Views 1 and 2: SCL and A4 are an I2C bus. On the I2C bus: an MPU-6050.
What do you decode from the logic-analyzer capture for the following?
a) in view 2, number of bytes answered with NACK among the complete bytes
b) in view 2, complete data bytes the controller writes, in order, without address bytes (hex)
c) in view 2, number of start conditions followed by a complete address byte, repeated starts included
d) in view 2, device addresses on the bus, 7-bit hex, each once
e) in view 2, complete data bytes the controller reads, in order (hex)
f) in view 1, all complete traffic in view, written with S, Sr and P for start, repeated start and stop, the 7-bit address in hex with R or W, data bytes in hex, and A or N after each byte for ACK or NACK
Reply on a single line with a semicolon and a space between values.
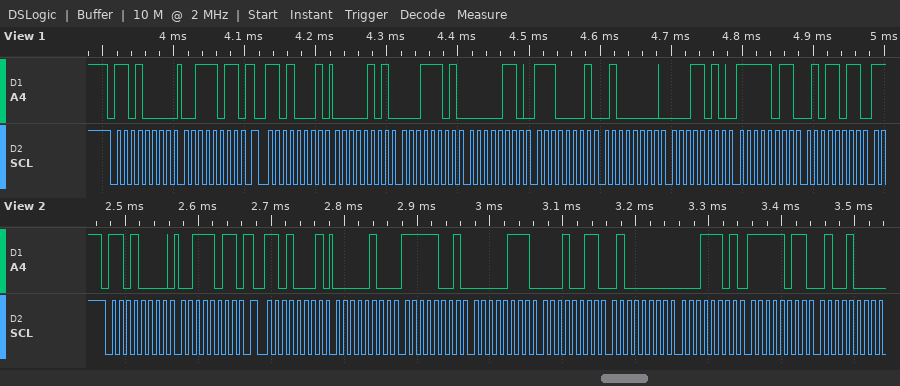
0; 3B; 2; 0x68; 04 F9 07 13 40 1D FB 48; S 68W A 3B A Sr 68R A 05 A 1D A 06 A E1 A 40 A 1A A FB A 5B A
